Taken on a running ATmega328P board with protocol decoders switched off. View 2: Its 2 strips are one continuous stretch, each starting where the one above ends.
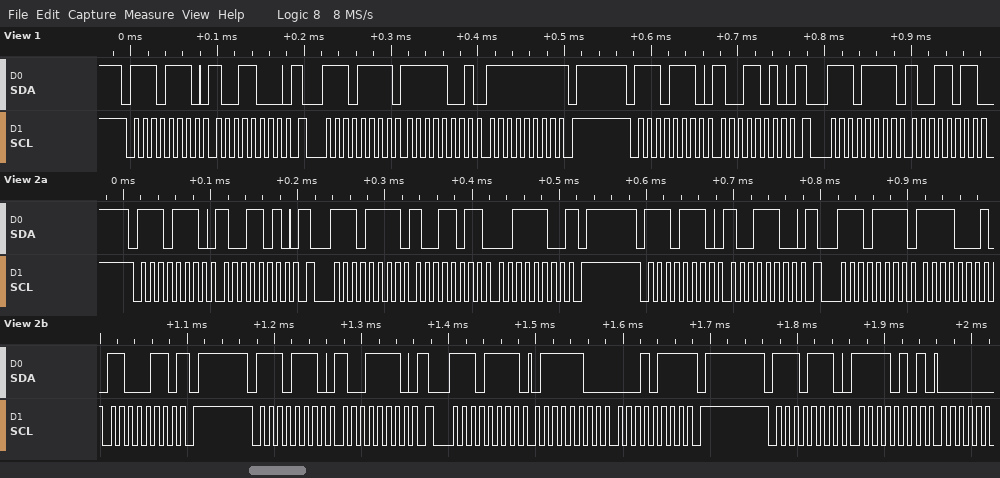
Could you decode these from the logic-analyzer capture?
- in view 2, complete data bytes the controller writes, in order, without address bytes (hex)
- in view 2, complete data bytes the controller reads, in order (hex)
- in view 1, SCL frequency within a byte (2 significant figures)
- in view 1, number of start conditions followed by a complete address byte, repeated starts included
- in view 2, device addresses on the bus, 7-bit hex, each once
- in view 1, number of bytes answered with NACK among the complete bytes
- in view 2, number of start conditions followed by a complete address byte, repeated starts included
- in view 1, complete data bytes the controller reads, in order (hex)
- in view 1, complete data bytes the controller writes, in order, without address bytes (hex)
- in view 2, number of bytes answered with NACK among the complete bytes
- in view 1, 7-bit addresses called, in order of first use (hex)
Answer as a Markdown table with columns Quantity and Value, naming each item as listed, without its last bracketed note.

| Quantity | Value |
|---|---|
| in view 2, complete data bytes the controller writes, in order, without address bytes | 9A 9C 9E F5 |
| in view 2, complete data bytes the controller reads, in order | 9B 3C F1 C6 7C 17 |
| in view 1, SCL frequency within a byte | 100 kHz |
| in view 1, number of start conditions followed by a complete address byte, repeated starts included | 4 |
| in view 2, device addresses on the bus, 7-bit hex, each once | 0x77 |
| in view 1, number of bytes answered with NACK among the complete bytes | 1 |
| in view 2, number of start conditions followed by a complete address byte, repeated starts included | 7 |
| in view 1, complete data bytes the controller reads, in order | F9 FF 9B |
| in view 1, complete data bytes the controller writes, in order, without address bytes | 98 9A |
| in view 2, number of bytes answered with NACK among the complete bytes | 3 |
| in view 1, 7-bit addresses called, in order of first use | 0x77 |
